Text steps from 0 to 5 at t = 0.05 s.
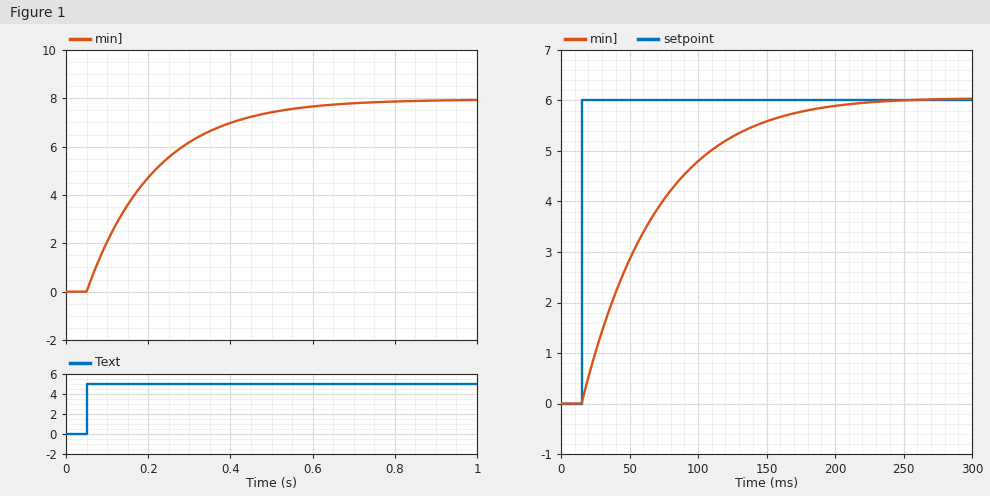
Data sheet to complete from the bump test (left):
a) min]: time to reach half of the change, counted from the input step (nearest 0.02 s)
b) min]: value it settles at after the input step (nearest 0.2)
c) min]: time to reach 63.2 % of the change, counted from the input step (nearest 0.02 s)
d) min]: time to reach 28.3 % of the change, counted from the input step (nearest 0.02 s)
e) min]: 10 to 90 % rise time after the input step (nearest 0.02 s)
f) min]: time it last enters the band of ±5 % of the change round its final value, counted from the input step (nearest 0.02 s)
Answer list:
0.12 s
8.0
0.16 s
0.06 s
0.36 s
0.50 s
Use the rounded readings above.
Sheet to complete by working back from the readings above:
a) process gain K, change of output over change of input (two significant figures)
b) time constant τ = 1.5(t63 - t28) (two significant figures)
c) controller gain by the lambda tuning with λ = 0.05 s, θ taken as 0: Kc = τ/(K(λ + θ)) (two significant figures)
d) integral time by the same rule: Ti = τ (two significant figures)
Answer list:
1.6
0.15 s
1.9
0.15 s
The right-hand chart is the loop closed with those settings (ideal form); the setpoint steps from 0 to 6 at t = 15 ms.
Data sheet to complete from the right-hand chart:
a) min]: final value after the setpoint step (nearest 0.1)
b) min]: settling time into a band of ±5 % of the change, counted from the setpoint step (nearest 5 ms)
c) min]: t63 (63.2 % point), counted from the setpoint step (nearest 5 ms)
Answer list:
6.0
150 ms
55 ms
